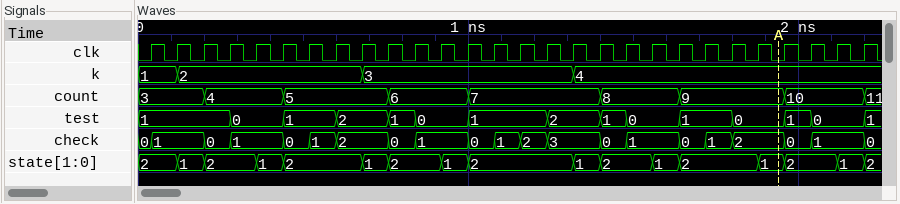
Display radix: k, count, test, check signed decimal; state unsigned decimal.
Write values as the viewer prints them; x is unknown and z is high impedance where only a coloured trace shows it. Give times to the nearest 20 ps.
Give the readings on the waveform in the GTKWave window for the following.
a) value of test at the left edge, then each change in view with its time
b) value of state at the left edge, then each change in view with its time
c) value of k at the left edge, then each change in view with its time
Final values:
1, 0 at 280 ps, 1 at 440 ps, 2 at 600 ps, 1 at 760 ps, 0 at 840 ps, 1 at 1000 ps, 2 at 1240 ps, 1 at 1400 ps, 0 at 1480 ps, 1 at 1640 ps, 0 at 1800 ps, 1 at 1960 ps, 0 at 2040 ps, 1 at 2200 ps
2, 1 at 120 ps, 2 at 200 ps, 1 at 360 ps, 2 at 440 ps, 1 at 680 ps, 2 at 760 ps, 1 at 920 ps, 2 at 1000 ps, 1 at 1320 ps, 2 at 1400 ps, 1 at 1560 ps, 2 at 1640 ps, 1 at 1880 ps, 2 at 1960 ps, 1 at 2120 ps, 2 at 2200 ps
1, 2 at 120 ps, 3 at 680 ps, 4 at 1320 ps
